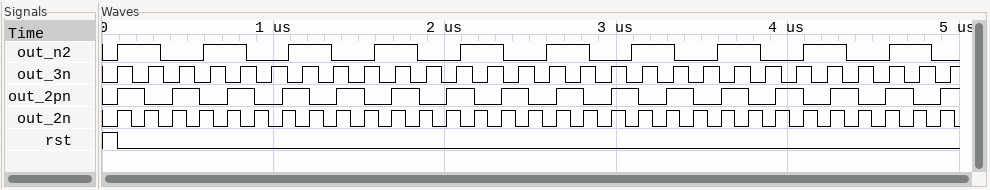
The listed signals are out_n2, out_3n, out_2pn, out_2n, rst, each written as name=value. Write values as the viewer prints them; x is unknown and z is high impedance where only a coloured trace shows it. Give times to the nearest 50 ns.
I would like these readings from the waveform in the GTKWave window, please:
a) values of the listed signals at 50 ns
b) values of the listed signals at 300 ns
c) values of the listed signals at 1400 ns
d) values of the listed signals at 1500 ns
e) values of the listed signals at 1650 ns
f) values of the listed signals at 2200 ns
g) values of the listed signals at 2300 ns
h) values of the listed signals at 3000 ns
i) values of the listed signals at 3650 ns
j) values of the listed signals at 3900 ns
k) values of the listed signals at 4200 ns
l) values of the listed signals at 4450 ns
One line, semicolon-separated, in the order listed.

out_n2=0, out_3n=0, out_2pn=0, out_2n=0, rst=1; out_n2=1, out_3n=1, out_2pn=0, out_2n=1, rst=0; out_n2=0, out_3n=1, out_2pn=1, out_2n=1, rst=0; out_n2=0, out_3n=0, out_2pn=1, out_2n=0, rst=0; out_n2=1, out_3n=0, out_2pn=0, out_2n=0, rst=0; out_n2=1, out_3n=0, out_2pn=0, out_2n=1, rst=0; out_n2=1, out_3n=1, out_2pn=0, out_2n=0, rst=0; out_n2=0, out_3n=1, out_2pn=1, out_2n=1, rst=0; out_n2=1, out_3n=0, out_2pn=1, out_2n=1, rst=0; out_n2=0, out_3n=1, out_2pn=0, out_2n=0, rst=0; out_n2=1, out_3n=0, out_2pn=0, out_2n=0, rst=0; out_n2=0, out_3n=1, out_2pn=0, out_2n=1, rst=0
